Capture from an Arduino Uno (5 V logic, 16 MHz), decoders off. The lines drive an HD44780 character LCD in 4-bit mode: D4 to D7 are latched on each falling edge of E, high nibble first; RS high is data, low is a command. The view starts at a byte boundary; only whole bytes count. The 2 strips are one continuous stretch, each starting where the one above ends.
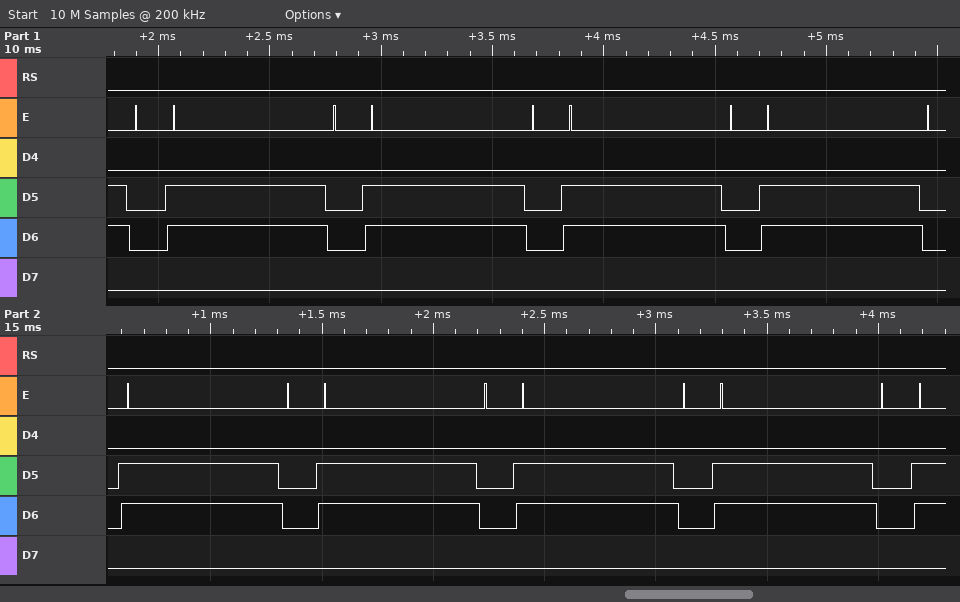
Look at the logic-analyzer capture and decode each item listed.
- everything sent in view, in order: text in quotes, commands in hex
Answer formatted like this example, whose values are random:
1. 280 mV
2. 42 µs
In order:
1. 0x06 0x06 0x06 0x06 0x06 0x06 0x06 0x06 0x06
